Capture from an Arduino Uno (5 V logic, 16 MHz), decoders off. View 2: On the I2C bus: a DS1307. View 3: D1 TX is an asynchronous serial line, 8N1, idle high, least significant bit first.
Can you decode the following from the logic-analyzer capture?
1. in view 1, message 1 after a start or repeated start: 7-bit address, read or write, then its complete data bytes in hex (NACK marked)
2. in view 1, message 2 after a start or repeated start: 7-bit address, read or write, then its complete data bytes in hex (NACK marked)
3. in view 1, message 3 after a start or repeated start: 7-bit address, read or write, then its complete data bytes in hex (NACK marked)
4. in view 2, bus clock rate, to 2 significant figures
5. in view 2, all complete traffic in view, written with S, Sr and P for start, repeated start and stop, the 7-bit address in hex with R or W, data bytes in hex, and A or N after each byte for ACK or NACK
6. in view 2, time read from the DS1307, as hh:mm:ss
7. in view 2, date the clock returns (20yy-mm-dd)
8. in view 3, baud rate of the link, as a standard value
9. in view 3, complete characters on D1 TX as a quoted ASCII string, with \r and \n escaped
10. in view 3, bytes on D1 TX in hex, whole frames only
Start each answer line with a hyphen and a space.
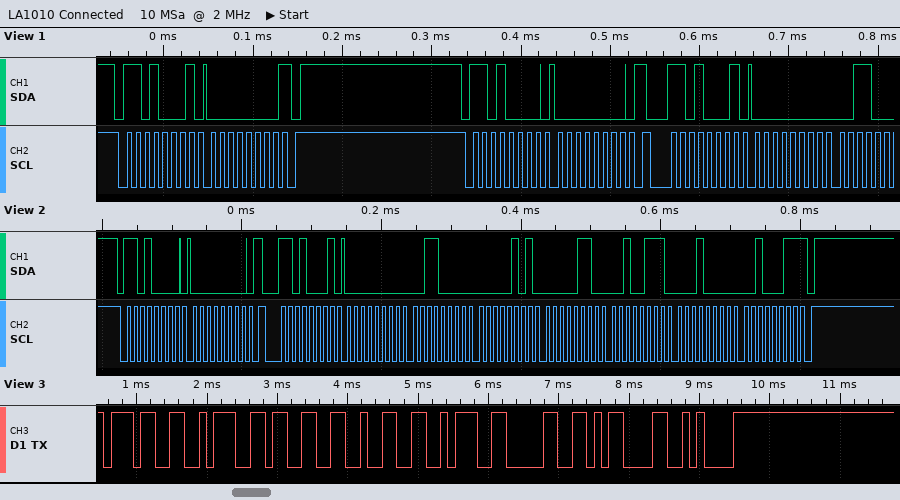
- 0x68 read: 00 NACK
- 0x68 write: 00
- 0x68 read: 00
- 100 kHz
- S 68W A 00 A Sr 68R A 00 A 30 A 05 A 06 A 27 A 10 A 23 N P
- 05:30:00
- 2023-10-27
- 9600 baud
- "7:32:0\r\n"
- 0x37 0x3A 0x33 0x32 0x3A 0x30 0x0D 0x0A
